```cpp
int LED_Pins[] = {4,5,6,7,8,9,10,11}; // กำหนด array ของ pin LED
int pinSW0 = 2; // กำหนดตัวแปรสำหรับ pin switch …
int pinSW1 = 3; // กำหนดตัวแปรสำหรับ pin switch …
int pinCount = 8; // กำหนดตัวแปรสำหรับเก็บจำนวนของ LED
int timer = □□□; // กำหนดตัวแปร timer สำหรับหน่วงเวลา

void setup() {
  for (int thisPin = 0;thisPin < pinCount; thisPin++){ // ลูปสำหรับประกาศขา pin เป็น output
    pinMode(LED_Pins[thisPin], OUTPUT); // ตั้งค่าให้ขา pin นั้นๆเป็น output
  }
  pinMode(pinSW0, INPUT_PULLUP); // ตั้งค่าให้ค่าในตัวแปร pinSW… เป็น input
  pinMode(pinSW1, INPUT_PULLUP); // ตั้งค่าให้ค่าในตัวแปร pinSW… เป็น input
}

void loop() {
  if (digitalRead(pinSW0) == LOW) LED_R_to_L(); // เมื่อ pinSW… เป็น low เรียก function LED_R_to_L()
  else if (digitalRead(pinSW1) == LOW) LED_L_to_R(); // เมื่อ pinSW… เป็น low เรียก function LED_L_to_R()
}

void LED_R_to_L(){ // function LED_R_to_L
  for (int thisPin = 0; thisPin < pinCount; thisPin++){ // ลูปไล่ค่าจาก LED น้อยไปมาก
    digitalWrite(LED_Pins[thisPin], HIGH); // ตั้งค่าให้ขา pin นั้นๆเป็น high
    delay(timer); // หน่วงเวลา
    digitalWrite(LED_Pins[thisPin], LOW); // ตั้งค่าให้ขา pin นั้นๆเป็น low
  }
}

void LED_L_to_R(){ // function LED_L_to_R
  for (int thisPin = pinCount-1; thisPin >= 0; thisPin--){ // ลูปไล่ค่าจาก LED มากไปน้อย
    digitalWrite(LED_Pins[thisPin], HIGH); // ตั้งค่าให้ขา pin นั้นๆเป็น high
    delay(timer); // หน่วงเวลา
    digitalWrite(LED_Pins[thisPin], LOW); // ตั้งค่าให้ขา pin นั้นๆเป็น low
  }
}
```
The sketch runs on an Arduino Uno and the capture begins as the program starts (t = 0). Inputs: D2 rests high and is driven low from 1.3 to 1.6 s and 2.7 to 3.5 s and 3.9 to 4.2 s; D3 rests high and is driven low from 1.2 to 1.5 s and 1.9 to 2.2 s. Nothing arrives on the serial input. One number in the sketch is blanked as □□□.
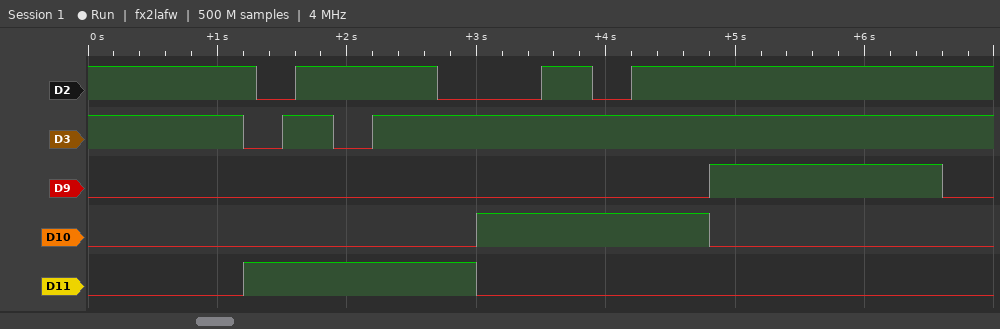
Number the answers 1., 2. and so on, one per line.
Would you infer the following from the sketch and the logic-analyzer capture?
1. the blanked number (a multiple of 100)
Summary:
1. 1800
